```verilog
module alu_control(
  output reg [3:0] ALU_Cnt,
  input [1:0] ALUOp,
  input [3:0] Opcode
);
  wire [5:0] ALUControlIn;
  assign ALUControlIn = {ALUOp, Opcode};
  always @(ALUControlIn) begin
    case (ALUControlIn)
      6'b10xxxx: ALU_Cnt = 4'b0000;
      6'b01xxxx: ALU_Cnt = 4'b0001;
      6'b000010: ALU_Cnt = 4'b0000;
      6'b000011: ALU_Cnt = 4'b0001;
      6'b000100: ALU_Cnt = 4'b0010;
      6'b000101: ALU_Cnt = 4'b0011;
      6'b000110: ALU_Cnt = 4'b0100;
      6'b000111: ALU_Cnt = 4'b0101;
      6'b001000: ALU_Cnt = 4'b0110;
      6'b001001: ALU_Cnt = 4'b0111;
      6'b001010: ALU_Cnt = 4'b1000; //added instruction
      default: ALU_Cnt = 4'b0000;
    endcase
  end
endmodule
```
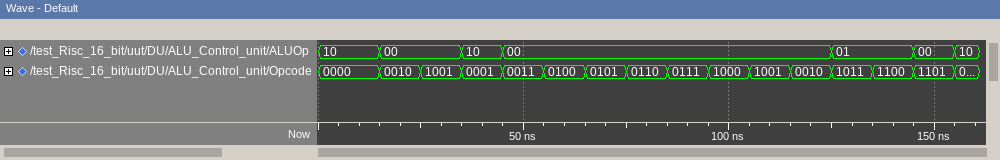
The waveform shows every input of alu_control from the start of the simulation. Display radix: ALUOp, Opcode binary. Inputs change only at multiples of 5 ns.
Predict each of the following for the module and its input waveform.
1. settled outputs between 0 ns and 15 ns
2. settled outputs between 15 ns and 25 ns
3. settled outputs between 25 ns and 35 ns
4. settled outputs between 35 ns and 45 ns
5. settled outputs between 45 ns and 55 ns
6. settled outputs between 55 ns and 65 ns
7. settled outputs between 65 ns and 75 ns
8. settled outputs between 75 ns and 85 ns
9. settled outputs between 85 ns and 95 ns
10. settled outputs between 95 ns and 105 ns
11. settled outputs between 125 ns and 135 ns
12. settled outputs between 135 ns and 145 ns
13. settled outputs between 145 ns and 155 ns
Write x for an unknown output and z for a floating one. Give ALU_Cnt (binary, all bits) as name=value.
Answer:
ALU_Cnt=0000
ALU_Cnt=0000
ALU_Cnt=0111
ALU_Cnt=0000
ALU_Cnt=0001
ALU_Cnt=0010
ALU_Cnt=0011
ALU_Cnt=0100
ALU_Cnt=0101
ALU_Cnt=0110
ALU_Cnt=0000
ALU_Cnt=0000
ALU_Cnt=0000
